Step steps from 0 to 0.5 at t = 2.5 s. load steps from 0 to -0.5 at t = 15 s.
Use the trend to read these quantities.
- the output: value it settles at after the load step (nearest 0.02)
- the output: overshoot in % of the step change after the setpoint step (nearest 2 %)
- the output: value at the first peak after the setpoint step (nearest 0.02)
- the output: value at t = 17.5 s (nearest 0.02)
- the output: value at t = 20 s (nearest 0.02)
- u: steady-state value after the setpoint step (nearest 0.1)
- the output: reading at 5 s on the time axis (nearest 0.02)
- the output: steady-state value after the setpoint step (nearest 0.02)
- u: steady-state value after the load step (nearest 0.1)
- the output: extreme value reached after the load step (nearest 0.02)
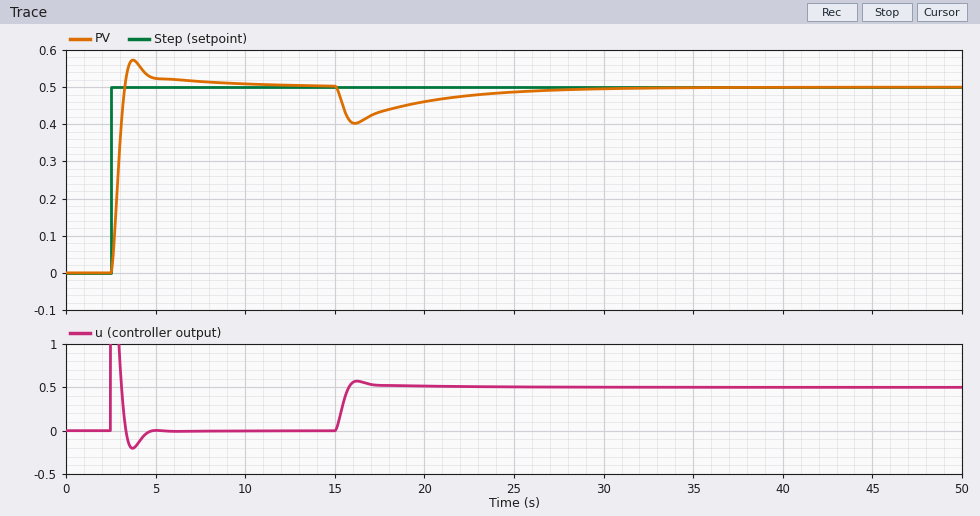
0.50
14 %
0.58
0.44
0.46
0.0
0.52
0.50
0.5
0.40
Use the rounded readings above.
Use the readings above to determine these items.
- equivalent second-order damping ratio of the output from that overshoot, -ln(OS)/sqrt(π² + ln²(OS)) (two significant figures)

0.53
